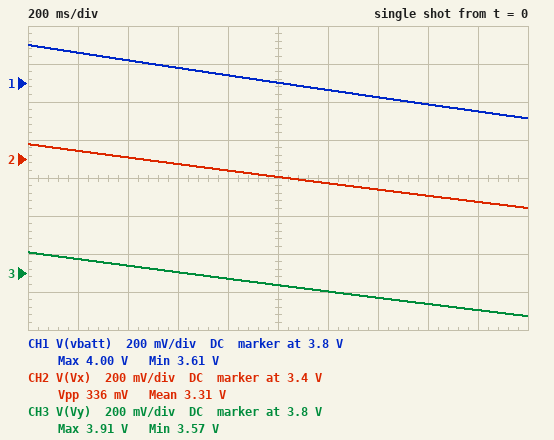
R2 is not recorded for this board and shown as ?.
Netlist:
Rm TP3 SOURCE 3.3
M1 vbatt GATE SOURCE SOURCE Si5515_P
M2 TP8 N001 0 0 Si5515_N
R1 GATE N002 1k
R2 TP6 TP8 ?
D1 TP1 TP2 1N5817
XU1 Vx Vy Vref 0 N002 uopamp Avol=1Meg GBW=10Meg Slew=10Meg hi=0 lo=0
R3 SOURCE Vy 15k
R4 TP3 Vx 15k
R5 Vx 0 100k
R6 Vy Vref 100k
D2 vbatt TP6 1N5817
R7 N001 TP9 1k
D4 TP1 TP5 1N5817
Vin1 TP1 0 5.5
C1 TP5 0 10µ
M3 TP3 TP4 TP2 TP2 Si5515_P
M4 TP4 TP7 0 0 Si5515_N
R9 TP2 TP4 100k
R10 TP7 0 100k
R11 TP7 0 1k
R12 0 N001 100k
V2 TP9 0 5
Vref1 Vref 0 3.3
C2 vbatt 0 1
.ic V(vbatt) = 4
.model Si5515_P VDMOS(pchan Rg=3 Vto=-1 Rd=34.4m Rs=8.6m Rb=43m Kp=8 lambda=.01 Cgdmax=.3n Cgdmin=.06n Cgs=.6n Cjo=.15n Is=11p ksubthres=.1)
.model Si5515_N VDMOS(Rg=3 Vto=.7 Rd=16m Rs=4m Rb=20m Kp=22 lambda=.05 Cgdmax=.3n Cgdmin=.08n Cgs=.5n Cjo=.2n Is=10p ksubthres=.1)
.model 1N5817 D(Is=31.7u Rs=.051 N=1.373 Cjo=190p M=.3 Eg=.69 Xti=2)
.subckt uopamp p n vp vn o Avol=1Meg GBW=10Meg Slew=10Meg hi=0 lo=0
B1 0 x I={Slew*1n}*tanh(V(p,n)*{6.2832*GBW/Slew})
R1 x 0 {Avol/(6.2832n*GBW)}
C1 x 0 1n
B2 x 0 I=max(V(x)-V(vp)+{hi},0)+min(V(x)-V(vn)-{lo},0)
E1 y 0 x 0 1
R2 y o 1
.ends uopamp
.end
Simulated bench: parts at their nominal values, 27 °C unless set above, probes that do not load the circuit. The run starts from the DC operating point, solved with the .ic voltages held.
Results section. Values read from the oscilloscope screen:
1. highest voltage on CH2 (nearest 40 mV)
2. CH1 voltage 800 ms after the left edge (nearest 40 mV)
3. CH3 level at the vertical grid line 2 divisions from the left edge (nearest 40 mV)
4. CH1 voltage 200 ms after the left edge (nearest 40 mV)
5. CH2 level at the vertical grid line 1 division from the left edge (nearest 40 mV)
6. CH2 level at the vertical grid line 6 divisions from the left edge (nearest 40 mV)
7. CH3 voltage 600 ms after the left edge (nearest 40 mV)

3.48 V
3.84 V
3.84 V
3.96 V
3.44 V
3.28 V
3.80 V
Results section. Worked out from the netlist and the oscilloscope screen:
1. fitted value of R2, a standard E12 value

18 Ω
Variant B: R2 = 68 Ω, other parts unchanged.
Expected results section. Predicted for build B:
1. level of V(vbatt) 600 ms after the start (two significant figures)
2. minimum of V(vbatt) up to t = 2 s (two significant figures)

4.0 V
3.9 V
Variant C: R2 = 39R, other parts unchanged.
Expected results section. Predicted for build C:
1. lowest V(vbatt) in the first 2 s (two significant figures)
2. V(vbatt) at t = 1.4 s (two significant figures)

3.8 V
3.9 V
